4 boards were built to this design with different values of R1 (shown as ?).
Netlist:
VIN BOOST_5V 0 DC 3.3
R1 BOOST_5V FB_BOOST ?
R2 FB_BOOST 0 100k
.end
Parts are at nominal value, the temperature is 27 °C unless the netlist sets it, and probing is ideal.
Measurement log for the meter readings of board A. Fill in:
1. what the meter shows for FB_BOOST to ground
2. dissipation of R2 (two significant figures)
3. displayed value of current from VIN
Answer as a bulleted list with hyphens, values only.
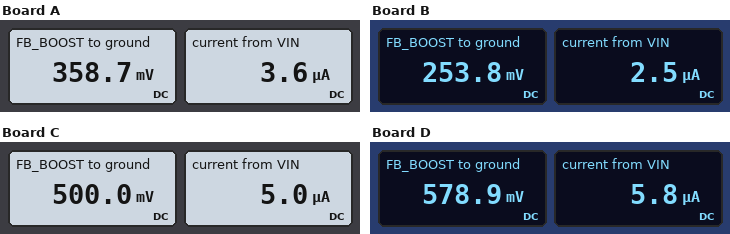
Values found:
- 358.7 mV
- 1.3 µW
- 3.6 µA
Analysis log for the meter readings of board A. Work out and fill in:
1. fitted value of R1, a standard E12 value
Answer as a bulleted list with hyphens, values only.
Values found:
- 820 kΩ
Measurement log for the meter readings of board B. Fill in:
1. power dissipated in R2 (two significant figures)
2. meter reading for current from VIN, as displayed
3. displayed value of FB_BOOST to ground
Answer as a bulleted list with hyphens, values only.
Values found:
- 640 nW
- 2.5 µA
- 253.8 mV
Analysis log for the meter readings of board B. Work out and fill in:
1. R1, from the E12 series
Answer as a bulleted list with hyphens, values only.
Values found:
- 1.2 MΩ
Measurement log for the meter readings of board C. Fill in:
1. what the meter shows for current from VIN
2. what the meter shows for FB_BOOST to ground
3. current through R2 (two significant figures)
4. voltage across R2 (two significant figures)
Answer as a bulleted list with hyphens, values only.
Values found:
- 5.0 µA
- 500.0 mV
- 5.0 µA
- 500 mV
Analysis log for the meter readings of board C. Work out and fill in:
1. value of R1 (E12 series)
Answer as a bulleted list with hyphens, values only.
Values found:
- 560 kΩ
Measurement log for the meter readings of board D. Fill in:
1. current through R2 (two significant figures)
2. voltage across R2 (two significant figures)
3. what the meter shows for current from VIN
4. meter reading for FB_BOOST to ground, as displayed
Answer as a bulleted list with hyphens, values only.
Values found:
- 5.8 µA
- 580 mV
- 5.8 µA
- 578.9 mV
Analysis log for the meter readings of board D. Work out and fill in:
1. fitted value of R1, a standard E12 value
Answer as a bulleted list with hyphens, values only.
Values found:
- 470 kΩ
